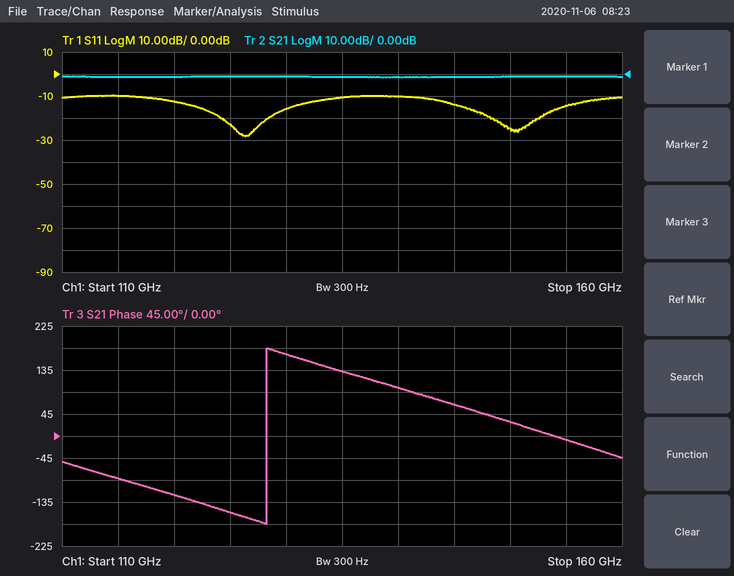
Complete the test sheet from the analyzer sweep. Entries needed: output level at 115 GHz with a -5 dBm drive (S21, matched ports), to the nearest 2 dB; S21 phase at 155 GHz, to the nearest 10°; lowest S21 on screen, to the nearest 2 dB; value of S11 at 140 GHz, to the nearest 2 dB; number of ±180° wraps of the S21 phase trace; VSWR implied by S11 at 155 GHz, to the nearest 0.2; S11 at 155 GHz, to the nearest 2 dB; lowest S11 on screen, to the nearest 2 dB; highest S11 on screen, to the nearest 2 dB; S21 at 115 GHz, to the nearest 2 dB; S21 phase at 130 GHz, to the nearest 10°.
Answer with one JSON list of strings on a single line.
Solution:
["-6 dBm", "-10°", "-2 dB", "-10 dB", "1", "1.4", "-14 dB", "-28 dB", "-10 dB", "-2 dB", "170°"]
